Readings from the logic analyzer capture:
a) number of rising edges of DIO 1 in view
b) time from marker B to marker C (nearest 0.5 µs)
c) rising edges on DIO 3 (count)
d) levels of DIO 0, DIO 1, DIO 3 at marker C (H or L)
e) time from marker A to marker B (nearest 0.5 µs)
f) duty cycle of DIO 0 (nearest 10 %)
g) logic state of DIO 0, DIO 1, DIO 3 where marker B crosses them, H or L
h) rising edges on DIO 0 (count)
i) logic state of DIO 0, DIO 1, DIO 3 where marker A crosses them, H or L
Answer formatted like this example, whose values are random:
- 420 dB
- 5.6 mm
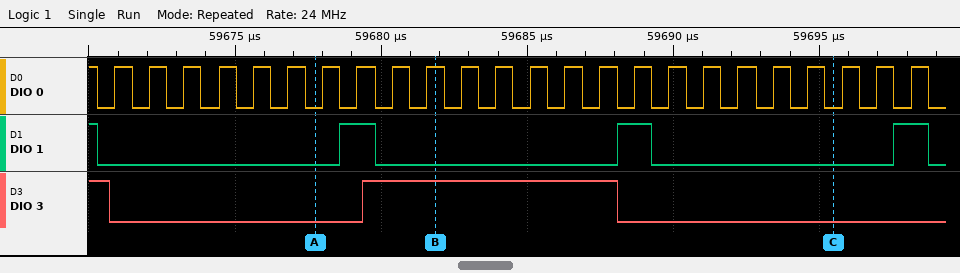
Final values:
- 3
- 13.5 µs
- 1
- DIO 0=L, DIO 1=L, DIO 3=L
- 4 µs
- 50 %
- DIO 0=H, DIO 1=L, DIO 3=H
- 24
- DIO 0=L, DIO 1=L, DIO 3=L
